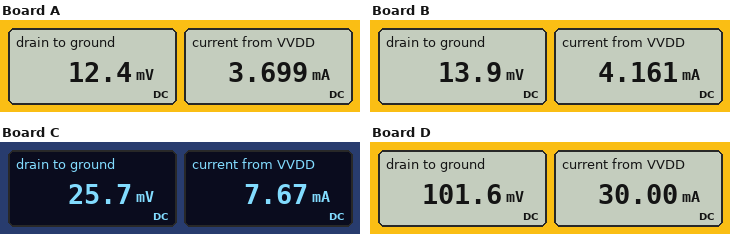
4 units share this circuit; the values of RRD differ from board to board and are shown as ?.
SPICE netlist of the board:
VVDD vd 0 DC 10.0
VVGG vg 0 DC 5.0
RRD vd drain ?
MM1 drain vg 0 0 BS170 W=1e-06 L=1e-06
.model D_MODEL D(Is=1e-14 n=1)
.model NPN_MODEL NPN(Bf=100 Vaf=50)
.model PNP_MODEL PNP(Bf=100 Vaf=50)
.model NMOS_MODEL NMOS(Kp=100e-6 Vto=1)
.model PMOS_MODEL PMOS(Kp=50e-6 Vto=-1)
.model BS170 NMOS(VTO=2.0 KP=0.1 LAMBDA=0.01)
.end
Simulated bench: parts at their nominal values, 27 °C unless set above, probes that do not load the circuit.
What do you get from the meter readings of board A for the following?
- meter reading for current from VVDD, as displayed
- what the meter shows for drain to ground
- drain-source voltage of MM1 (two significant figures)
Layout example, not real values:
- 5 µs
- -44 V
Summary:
- 3.699 mA
- 12.4 mV
- 12 mV
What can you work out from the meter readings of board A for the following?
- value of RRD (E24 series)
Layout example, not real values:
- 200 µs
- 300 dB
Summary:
- 2.7 kΩ
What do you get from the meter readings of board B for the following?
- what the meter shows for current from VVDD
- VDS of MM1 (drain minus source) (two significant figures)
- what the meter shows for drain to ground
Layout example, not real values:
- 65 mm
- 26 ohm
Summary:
- 4.161 mA
- 14 mV
- 13.9 mV
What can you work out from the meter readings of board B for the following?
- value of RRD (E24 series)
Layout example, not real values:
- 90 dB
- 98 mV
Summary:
- 2.4 kΩ
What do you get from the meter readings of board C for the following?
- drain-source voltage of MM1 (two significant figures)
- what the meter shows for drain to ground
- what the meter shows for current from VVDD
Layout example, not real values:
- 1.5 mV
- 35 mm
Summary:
- 26 mV
- 25.7 mV
- 7.67 mA
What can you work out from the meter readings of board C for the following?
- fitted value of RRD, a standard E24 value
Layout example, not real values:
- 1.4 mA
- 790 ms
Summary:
- 1.3 kΩ
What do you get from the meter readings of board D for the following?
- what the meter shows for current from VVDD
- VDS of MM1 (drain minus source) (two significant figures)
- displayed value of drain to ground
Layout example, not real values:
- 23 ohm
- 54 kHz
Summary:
- 30.00 mA
- 100 mV
- 101.6 mV
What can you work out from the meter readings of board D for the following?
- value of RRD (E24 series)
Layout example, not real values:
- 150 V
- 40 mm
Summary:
- 330 Ω
